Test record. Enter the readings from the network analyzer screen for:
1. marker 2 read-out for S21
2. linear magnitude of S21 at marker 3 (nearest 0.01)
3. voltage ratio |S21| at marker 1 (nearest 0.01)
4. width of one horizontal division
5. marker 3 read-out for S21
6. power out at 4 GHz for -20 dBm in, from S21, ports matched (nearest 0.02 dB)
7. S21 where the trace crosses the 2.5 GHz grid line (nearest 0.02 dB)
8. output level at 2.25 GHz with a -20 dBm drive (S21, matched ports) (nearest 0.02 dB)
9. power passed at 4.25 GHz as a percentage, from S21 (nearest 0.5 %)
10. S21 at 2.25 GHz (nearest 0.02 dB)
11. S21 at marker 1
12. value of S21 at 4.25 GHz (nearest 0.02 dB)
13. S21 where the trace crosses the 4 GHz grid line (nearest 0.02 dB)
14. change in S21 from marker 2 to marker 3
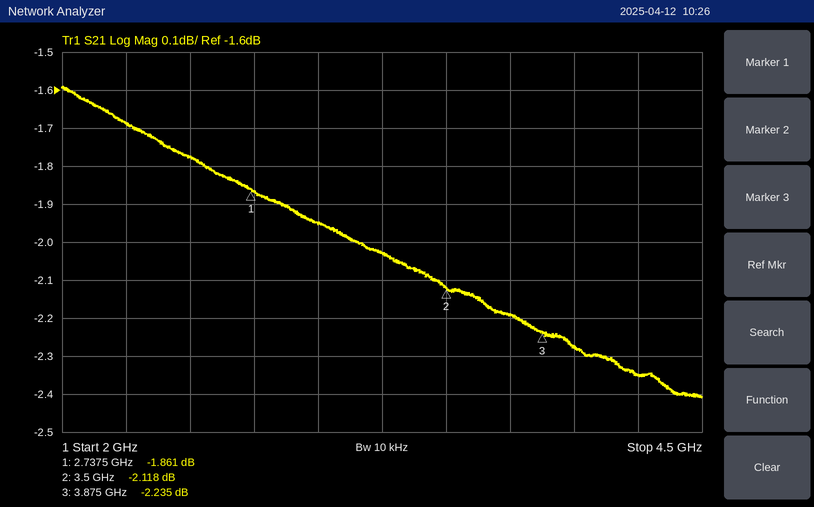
-2.118 dB
0.77
0.81
250 MHz
-2.235 dB
-22.28 dBm
-1.78 dB
-21.68 dBm
58.0 %
-1.68 dB
-1.861 dB
-2.36 dB
-2.28 dB
-0.117 dB
